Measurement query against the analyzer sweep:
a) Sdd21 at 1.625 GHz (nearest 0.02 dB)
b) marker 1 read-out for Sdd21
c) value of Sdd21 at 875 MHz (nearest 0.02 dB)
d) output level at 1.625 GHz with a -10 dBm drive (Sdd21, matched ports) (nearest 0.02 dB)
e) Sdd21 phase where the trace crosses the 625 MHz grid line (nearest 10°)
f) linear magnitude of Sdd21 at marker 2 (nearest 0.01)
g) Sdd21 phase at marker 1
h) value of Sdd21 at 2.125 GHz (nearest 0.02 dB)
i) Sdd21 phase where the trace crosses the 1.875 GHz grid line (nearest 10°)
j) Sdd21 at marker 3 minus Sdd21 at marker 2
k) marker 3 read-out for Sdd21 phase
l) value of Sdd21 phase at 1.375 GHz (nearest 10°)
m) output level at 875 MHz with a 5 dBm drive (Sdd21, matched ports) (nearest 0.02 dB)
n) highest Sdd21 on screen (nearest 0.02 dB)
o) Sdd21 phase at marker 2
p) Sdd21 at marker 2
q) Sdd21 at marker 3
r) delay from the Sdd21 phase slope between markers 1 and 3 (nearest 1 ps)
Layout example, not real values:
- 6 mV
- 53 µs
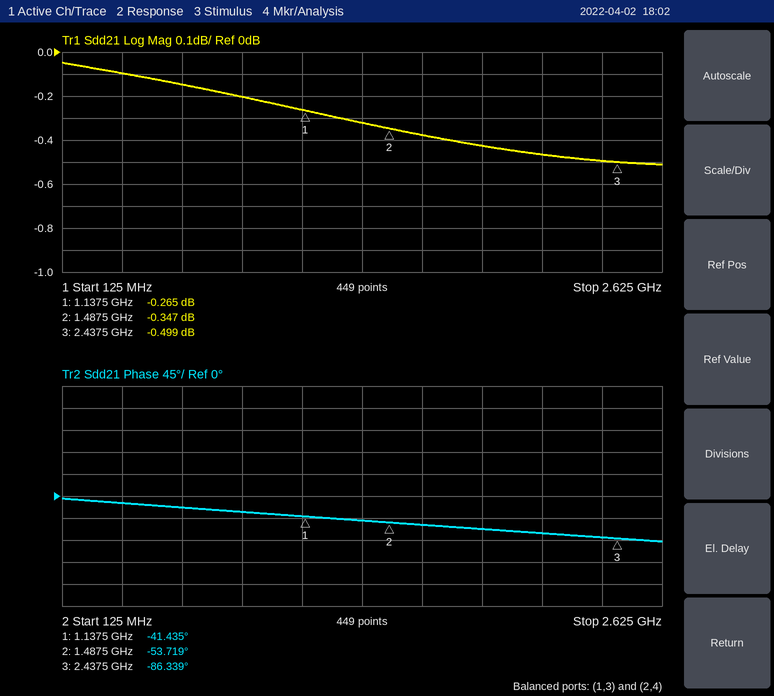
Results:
- -0.38 dB
- -0.265 dB
- -0.20 dB
- -10.38 dBm
- -20°
- 0.96
- -41.435°
- -0.46 dB
- -70°
- -0.152 dB
- -86.339°
- -50°
- 4.80 dBm
- -0.04 dB
- -53.719°
- -0.347 dB
- -0.499 dB
- 96 ps
